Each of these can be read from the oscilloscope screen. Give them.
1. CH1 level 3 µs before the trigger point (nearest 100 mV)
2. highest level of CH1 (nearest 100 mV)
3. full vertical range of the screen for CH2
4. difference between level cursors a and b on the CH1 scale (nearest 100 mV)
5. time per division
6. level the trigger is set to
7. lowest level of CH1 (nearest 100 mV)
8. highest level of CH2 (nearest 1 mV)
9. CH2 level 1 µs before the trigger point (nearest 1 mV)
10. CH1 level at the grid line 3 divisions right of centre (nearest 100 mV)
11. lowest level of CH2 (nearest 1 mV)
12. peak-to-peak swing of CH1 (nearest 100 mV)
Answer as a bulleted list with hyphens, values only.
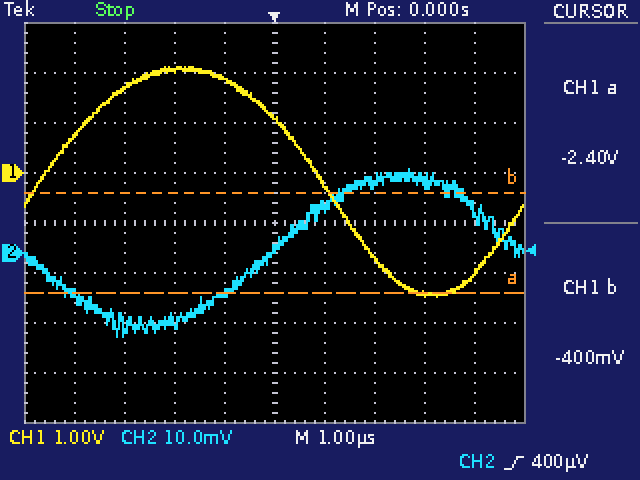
- 1.7 V
- 2.1 V
- 80 mV
- 2.0 V
- 1 µs
- 400 µV
- -2.5 V
- 17 mV
- -8 mV
- -2.4 V
- -17 mV
- 4.6 V
